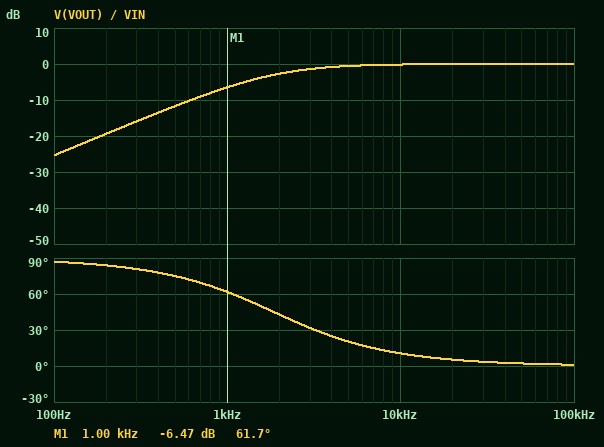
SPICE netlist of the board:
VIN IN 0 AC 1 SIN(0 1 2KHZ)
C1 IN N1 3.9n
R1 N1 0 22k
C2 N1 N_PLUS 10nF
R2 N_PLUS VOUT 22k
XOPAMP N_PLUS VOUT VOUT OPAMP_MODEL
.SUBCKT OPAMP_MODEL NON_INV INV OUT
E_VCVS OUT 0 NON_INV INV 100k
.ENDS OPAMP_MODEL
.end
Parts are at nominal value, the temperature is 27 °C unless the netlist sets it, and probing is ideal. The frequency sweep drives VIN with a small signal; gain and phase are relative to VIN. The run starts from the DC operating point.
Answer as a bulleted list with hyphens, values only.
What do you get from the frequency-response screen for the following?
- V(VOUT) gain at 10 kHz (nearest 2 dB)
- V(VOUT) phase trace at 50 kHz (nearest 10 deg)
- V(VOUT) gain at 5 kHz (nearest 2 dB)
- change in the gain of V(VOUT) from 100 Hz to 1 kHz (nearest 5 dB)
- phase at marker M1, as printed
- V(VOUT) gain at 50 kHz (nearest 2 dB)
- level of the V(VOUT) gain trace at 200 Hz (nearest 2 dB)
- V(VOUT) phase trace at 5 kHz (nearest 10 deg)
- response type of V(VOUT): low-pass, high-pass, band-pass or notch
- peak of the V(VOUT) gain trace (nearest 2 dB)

- 0 dB
- 0 deg
- 0 dB
- 20 dB
- 61.7 deg
- 0 dB
- -20 dB
- 20 deg
- high-pass
- 0 dB
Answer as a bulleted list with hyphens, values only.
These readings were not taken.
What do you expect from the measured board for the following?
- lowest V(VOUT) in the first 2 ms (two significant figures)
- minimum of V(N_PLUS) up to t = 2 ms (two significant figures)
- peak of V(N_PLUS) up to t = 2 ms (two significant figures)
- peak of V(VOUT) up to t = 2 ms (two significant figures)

- -750 mV
- -750 mV
- 730 mV
- 730 mV
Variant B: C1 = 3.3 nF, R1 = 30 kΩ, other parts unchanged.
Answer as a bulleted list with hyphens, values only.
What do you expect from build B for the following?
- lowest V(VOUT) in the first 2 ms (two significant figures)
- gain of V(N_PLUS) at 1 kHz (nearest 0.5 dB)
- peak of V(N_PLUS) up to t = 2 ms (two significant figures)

- -800 mV
- -5.5 dB
- 780 mV
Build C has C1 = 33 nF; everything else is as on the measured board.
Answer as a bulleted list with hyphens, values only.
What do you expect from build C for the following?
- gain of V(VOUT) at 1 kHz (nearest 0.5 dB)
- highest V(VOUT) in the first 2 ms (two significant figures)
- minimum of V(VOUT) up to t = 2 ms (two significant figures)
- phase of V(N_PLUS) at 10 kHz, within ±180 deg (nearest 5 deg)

- 0 dB
- 980 mV
- -1.1 V
- 0 deg
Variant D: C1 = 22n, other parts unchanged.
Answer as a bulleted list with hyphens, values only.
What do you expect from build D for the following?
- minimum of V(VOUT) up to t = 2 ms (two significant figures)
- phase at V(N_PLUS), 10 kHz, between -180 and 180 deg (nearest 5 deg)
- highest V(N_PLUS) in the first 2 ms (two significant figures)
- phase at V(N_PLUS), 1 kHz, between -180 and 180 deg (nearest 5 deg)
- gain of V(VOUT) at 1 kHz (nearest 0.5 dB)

- -1.1 V
- 0 deg
- 980 mV
- 20 deg
- -0.5 dB
